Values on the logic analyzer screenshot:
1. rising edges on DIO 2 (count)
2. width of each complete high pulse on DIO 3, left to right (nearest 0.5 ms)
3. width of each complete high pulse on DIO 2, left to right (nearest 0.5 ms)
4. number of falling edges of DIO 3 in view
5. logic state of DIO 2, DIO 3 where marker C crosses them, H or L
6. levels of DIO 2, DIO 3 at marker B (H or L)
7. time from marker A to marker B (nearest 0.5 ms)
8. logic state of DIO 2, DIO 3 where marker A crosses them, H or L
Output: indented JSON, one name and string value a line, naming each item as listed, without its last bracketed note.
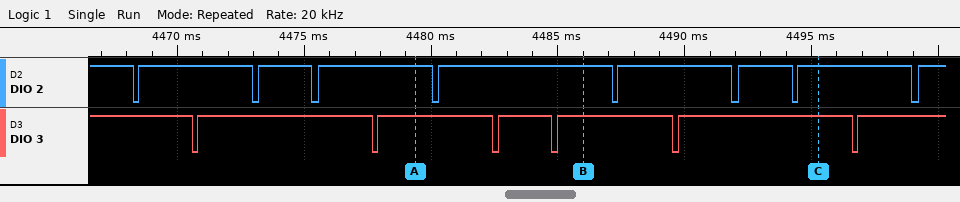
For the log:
{
  "rising edges on DIO 2": "8",
  "width of each complete high pulse on DIO 3, left to right": "7 ms, 4.5 ms, 2 ms, 4.5 ms, 7 ms",
  "width of each complete high pulse on DIO 2, left to right": "4.5 ms, 2 ms, 4.5 ms, 7 ms, 4.5 ms, 2 ms, 4.5 ms",
  "number of falling edges of DIO 3 in view": "6",
  "logic state of DIO 2, DIO 3 where marker C crosses them, H or L": "DIO 2=H, DIO 3=H",
  "levels of DIO 2, DIO 3 at marker B": "DIO 2=H, DIO 3=H",
  "time from marker A to marker B": "6.5 ms",
  "logic state of DIO 2, DIO 3 where marker A crosses them, H or L": "DIO 2=H, DIO 3=H"
}
